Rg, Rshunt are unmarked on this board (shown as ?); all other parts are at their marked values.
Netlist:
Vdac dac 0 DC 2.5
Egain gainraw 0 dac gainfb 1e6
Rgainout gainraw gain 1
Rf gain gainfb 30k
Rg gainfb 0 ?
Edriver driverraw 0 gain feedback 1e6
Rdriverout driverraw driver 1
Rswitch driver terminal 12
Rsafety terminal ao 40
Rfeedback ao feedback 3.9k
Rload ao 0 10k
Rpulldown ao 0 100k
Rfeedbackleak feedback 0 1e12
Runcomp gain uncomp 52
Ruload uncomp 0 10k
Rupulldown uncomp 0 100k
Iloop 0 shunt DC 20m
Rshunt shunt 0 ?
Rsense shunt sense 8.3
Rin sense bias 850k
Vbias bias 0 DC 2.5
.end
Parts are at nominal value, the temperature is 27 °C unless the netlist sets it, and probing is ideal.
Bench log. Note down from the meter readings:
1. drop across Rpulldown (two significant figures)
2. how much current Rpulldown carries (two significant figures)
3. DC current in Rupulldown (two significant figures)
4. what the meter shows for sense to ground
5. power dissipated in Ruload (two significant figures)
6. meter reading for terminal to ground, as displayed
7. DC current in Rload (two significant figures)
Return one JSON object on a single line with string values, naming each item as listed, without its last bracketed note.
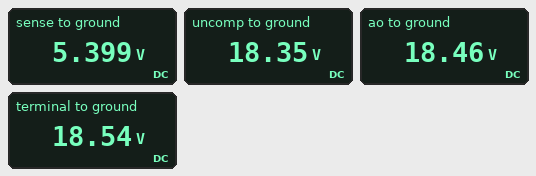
{"drop across Rpulldown": "18 V", "how much current Rpulldown carries": "180 µA", "DC current in Rupulldown": "180 µA", "what the meter shows for sense to ground": "5.399 V", "power dissipated in Ruload": "34 mW", "meter reading for terminal to ground, as displayed": "18.54 V", "DC current in Rload": "1.8 mA"}
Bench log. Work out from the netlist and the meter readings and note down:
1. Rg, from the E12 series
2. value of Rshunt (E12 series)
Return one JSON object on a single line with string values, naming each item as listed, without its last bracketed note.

{"Rg, from the E12 series": "4.7 kΩ", "value of Rshunt": "270 Ω"}
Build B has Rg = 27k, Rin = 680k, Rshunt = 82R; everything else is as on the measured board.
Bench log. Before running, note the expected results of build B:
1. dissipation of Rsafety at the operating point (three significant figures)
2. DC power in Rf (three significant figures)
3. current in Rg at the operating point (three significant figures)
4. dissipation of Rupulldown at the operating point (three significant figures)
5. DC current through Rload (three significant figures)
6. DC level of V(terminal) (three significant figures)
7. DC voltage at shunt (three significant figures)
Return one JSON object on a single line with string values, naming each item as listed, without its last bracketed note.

{"dissipation of Rsafety at the operating point": "13.5 µW", "DC power in Rf": "257 µW", "current in Rg at the operating point": "92.6 µA", "dissipation of Rupulldown at the operating point": "275 µW", "DC current through Rload": "528 µA", "DC level of V(terminal)": "5.30 V", "DC voltage at shunt": "1.64 V"}
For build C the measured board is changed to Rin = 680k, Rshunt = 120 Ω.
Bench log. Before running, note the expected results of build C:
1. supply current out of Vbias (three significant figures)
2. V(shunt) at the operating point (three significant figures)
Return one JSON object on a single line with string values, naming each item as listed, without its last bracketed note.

{"supply current out of Vbias": "147 nA", "V(shunt) at the operating point": "2.40 V"}
